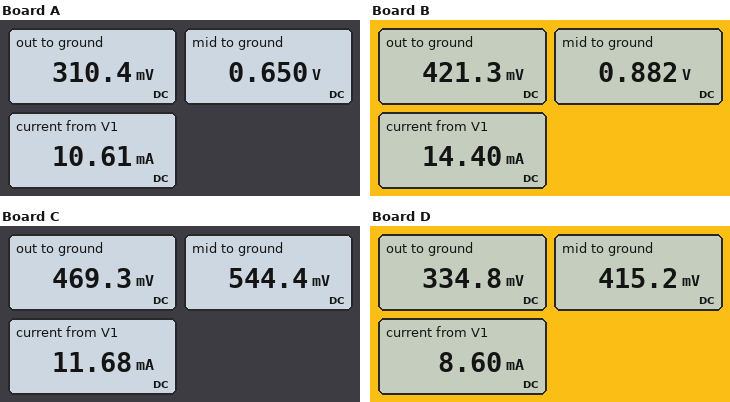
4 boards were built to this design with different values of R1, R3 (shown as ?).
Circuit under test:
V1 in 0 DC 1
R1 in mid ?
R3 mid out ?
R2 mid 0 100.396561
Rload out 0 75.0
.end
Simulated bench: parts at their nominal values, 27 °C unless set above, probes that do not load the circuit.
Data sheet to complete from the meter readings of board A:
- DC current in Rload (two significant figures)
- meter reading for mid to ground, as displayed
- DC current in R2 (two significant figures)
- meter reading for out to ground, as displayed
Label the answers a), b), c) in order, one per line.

a) 4.1 mA
b) 0.650 V
c) 6.5 mA
d) 310.4 mV
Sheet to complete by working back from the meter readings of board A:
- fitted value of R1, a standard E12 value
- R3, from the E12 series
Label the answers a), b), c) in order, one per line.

a) 33 Ω
b) 82 Ω
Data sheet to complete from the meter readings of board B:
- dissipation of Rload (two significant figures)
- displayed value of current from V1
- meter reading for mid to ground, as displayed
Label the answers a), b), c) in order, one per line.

a) 2.4 mW
b) 14.40 mA
c) 0.882 V
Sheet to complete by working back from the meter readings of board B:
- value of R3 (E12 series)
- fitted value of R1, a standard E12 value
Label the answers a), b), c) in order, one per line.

a) 82 Ω
b) 8.2 Ω
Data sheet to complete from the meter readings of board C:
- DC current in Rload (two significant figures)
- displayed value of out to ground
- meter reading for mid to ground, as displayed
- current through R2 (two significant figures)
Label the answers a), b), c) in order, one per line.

a) 6.3 mA
b) 469.3 mV
c) 544.4 mV
d) 5.4 mA
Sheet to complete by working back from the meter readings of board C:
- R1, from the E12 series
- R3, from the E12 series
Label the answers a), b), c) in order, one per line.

a) 39 Ω
b) 12 Ω
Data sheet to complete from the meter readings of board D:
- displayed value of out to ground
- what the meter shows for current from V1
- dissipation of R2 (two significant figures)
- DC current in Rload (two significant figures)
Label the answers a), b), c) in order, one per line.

a) 334.8 mV
b) 8.60 mA
c) 1.7 mW
d) 4.5 mA
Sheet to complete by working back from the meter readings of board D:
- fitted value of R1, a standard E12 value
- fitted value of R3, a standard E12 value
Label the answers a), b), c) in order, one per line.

a) 68 Ω
b) 18 Ω
